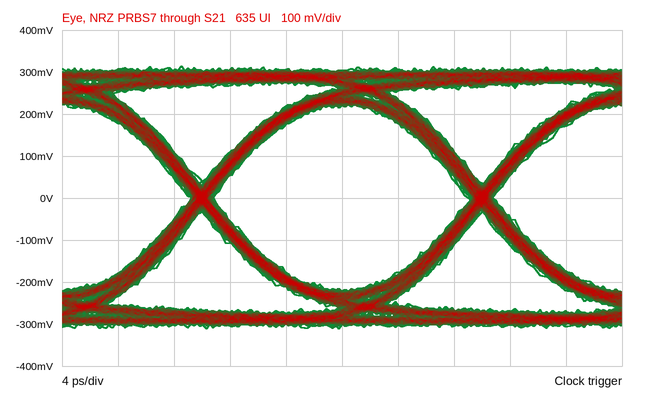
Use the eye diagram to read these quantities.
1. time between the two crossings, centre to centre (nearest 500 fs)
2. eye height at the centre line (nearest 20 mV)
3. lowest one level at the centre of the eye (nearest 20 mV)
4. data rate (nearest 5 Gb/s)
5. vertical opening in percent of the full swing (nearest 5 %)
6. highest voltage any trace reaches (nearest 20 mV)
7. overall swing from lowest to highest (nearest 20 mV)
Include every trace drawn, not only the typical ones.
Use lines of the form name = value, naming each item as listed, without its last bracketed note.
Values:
time between the two crossings, centre to centre = 20.0 ps
eye height at the centre line = 440 mV
lowest one level at the centre of the eye = 220 mV
data rate = 50 Gb/s
vertical opening in percent of the full swing = 70 %
highest voltage any trace reaches = 320 mV
overall swing from lowest to highest = 620 mV
